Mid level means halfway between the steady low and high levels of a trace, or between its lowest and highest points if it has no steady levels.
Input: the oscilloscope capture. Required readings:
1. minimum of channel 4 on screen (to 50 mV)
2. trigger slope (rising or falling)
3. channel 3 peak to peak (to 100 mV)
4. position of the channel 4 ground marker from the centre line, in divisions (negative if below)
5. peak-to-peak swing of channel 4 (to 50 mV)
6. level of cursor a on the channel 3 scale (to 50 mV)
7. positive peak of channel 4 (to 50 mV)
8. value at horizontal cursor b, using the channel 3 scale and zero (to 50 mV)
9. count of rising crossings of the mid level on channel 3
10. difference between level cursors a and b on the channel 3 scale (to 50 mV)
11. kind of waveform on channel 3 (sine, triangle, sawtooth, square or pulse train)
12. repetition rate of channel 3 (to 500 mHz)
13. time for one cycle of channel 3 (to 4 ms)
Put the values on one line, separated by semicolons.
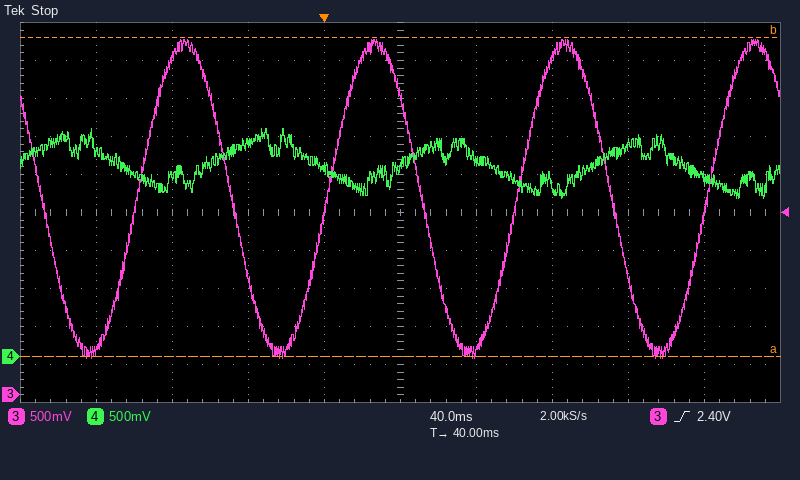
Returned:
2.10 V; rising; 4.20 V; -3.8 div; 900 mV; 500 mV; 3.00 V; 4.70 V; 4; 4.20 V; sine; 10.0 Hz; 100 ms
